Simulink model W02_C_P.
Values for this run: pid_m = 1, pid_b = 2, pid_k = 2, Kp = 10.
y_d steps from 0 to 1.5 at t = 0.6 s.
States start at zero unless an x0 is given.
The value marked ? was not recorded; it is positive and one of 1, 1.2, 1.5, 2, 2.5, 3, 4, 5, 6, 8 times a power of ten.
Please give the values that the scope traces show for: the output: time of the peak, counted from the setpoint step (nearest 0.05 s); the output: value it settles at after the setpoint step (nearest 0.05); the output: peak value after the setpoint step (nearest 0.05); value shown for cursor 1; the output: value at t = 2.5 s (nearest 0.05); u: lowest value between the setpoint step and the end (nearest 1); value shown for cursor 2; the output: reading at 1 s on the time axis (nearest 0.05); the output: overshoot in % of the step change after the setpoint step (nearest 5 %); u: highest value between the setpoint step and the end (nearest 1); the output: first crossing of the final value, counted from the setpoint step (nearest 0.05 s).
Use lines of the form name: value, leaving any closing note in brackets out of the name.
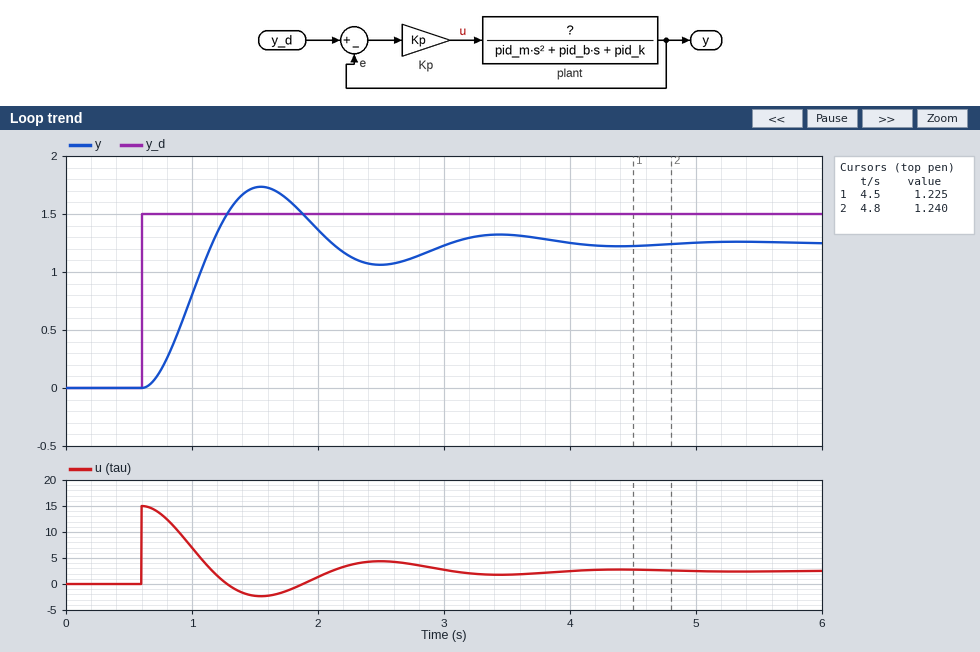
the output: time of the peak, counted from the setpoint step: 0.95 s
the output: value it settles at after the setpoint step: 1.25
the output: peak value after the setpoint step: 1.75
value shown for cursor 1: 1.225
the output: value at t = 2.5 s: 1.05
u: lowest value between the setpoint step and the end: -2
value shown for cursor 2: 1.240
the output: reading at 1 s on the time axis: 0.80
the output: overshoot in % of the step change after the setpoint step: 40 %
u: highest value between the setpoint step and the end: 15
the output: first crossing of the final value, counted from the setpoint step: 0.55 s
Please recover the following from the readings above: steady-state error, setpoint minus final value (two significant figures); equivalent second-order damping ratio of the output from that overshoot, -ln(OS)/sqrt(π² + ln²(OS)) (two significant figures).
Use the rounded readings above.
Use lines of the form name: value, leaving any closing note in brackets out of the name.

steady-state error, setpoint minus final value: 0.25
equivalent second-order damping ratio of the output from that overshoot, -ln(OS)/sqrt(π² + ln²(OS)): 0.28
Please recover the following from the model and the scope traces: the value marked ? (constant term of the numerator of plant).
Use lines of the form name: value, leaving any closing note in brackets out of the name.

the value marked ?: 1
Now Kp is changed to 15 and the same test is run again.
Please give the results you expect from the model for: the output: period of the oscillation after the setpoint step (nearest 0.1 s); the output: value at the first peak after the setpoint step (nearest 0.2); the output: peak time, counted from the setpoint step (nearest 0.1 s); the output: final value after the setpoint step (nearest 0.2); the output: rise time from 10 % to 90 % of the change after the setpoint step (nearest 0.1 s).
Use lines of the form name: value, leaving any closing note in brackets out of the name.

the output: period of the oscillation after the setpoint step: 1.6 s
the output: value at the first peak after the setpoint step: 2.0
the output: peak time, counted from the setpoint step: 0.8 s
the output: final value after the setpoint step: 1.4
the output: rise time from 10 % to 90 % of the change after the setpoint step: 0.3 s
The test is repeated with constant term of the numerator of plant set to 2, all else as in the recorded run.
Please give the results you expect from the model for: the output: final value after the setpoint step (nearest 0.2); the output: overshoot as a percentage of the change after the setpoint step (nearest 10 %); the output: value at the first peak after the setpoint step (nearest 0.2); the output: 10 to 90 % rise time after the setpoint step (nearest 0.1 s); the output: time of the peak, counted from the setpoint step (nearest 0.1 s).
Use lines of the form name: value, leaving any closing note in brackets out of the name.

the output: final value after the setpoint step: 1.4
the output: overshoot as a percentage of the change after the setpoint step: 50 %
the output: value at the first peak after the setpoint step: 2.0
the output: 10 to 90 % rise time after the setpoint step: 0.3 s
the output: time of the peak, counted from the setpoint step: 0.7 s
